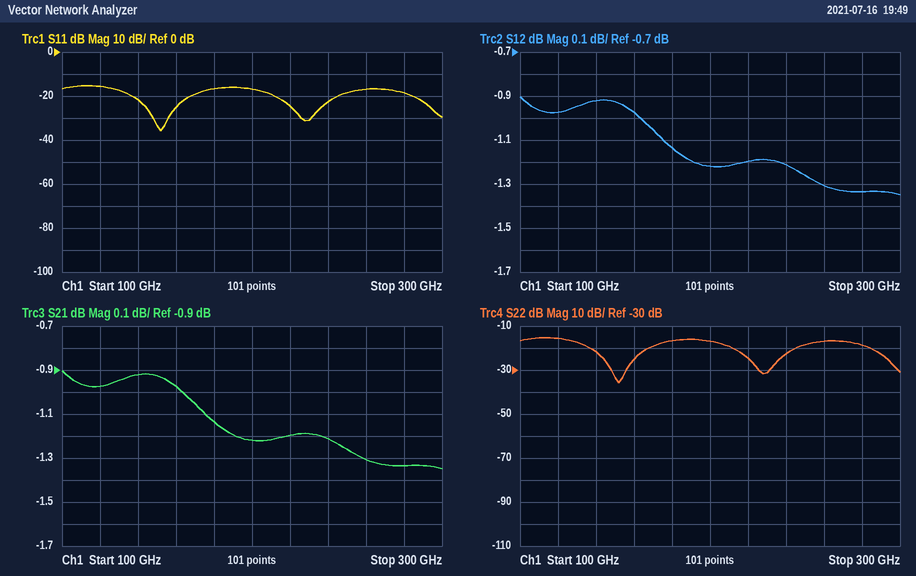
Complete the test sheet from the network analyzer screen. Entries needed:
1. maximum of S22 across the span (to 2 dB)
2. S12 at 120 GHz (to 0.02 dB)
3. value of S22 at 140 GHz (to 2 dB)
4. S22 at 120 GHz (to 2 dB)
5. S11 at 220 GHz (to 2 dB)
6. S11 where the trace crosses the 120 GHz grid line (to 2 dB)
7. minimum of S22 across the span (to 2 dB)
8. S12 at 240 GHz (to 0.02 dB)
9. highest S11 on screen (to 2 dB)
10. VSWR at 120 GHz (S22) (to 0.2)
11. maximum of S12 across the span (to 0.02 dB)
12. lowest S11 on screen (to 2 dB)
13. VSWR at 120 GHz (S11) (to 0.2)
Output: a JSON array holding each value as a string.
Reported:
["-16 dB", "-0.98 dB", "-22 dB", "-16 dB", "-24 dB", "-16 dB", "-36 dB", "-1.22 dB", "-16 dB", "1.4", "-0.90 dB", "-36 dB", "1.4"]
